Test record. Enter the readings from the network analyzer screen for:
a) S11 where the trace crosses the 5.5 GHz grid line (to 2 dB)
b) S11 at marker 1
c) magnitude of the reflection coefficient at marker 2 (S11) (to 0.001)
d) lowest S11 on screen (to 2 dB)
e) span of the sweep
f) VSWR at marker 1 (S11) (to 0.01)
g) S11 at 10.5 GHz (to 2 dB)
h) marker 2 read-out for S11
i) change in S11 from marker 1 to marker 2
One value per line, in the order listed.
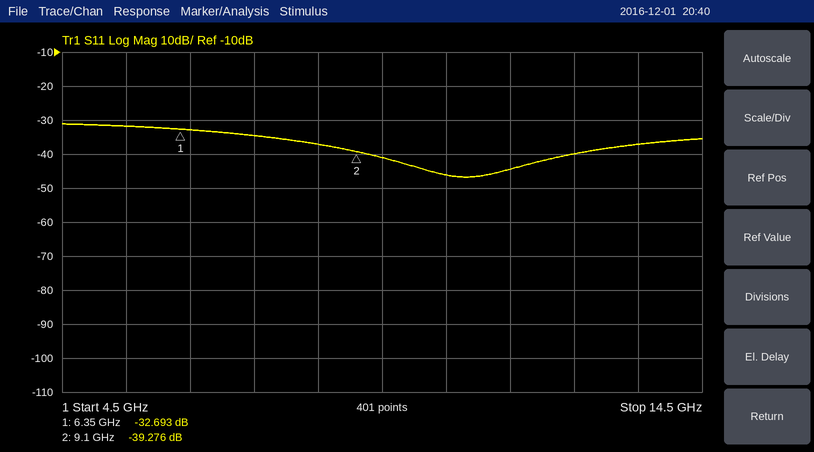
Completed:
-32 dB
-32.693 dB
0.011
-46 dB
10 GHz
1.05
-46 dB
-39.276 dB
-6.583 dB
